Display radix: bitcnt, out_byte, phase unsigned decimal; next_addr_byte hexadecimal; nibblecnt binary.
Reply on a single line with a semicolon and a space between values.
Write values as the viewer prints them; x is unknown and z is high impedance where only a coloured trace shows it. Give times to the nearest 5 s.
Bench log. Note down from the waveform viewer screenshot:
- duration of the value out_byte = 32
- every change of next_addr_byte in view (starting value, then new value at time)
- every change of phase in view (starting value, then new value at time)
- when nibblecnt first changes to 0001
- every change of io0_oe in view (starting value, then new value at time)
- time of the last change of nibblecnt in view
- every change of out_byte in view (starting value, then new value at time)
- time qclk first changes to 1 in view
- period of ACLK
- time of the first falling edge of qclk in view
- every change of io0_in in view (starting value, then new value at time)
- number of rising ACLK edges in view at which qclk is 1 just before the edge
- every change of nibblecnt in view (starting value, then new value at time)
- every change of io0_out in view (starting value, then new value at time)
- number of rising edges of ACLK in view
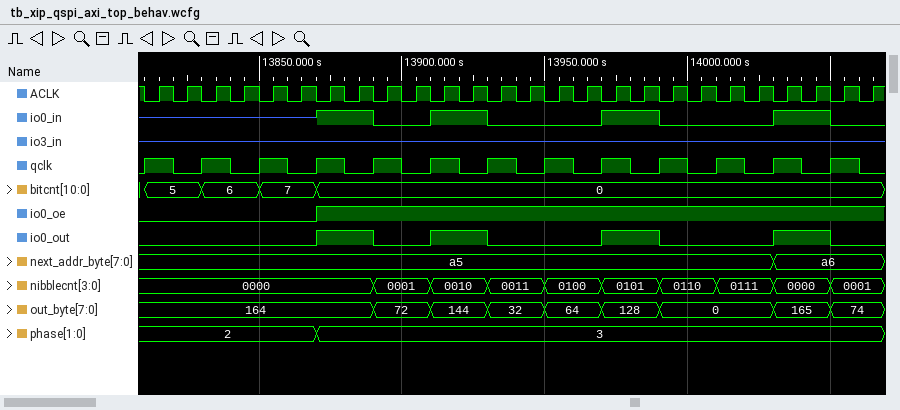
20 s; a5, a6 at 14030 s; 2, 3 at 13870 s; 13890 s; 0, 1 at 13870 s; 14050 s; 164, 72 at 13890 s, 144 at 13910 s, 32 at 13930 s, 64 at 13950 s, 128 at 13970 s, 0 at 13990 s, 165 at 14030 s, 74 at 14050 s; 13810 s; 10 s; 13820 s; z, 1 at 13870 s, 0 at 13890 s, 1 at 13910 s, 0 at 13930 s, 1 at 13970 s, 0 at 13990 s, 1 at 14030 s, 0 at 14050 s; 13; 0000, 0001 at 13890 s, 0010 at 13910 s, 0011 at 13930 s, 0100 at 13950 s, 0101 at 13970 s, 0110 at 13990 s, 0111 at 14010 s, 0000 at 14030 s, 0001 at 14050 s; 0, 1 at 13870 s, 0 at 13890 s, 1 at 13910 s, 0 at 13930 s, 1 at 13970 s, 0 at 13990 s, 1 at 14030 s, 0 at 14050 s; 26
